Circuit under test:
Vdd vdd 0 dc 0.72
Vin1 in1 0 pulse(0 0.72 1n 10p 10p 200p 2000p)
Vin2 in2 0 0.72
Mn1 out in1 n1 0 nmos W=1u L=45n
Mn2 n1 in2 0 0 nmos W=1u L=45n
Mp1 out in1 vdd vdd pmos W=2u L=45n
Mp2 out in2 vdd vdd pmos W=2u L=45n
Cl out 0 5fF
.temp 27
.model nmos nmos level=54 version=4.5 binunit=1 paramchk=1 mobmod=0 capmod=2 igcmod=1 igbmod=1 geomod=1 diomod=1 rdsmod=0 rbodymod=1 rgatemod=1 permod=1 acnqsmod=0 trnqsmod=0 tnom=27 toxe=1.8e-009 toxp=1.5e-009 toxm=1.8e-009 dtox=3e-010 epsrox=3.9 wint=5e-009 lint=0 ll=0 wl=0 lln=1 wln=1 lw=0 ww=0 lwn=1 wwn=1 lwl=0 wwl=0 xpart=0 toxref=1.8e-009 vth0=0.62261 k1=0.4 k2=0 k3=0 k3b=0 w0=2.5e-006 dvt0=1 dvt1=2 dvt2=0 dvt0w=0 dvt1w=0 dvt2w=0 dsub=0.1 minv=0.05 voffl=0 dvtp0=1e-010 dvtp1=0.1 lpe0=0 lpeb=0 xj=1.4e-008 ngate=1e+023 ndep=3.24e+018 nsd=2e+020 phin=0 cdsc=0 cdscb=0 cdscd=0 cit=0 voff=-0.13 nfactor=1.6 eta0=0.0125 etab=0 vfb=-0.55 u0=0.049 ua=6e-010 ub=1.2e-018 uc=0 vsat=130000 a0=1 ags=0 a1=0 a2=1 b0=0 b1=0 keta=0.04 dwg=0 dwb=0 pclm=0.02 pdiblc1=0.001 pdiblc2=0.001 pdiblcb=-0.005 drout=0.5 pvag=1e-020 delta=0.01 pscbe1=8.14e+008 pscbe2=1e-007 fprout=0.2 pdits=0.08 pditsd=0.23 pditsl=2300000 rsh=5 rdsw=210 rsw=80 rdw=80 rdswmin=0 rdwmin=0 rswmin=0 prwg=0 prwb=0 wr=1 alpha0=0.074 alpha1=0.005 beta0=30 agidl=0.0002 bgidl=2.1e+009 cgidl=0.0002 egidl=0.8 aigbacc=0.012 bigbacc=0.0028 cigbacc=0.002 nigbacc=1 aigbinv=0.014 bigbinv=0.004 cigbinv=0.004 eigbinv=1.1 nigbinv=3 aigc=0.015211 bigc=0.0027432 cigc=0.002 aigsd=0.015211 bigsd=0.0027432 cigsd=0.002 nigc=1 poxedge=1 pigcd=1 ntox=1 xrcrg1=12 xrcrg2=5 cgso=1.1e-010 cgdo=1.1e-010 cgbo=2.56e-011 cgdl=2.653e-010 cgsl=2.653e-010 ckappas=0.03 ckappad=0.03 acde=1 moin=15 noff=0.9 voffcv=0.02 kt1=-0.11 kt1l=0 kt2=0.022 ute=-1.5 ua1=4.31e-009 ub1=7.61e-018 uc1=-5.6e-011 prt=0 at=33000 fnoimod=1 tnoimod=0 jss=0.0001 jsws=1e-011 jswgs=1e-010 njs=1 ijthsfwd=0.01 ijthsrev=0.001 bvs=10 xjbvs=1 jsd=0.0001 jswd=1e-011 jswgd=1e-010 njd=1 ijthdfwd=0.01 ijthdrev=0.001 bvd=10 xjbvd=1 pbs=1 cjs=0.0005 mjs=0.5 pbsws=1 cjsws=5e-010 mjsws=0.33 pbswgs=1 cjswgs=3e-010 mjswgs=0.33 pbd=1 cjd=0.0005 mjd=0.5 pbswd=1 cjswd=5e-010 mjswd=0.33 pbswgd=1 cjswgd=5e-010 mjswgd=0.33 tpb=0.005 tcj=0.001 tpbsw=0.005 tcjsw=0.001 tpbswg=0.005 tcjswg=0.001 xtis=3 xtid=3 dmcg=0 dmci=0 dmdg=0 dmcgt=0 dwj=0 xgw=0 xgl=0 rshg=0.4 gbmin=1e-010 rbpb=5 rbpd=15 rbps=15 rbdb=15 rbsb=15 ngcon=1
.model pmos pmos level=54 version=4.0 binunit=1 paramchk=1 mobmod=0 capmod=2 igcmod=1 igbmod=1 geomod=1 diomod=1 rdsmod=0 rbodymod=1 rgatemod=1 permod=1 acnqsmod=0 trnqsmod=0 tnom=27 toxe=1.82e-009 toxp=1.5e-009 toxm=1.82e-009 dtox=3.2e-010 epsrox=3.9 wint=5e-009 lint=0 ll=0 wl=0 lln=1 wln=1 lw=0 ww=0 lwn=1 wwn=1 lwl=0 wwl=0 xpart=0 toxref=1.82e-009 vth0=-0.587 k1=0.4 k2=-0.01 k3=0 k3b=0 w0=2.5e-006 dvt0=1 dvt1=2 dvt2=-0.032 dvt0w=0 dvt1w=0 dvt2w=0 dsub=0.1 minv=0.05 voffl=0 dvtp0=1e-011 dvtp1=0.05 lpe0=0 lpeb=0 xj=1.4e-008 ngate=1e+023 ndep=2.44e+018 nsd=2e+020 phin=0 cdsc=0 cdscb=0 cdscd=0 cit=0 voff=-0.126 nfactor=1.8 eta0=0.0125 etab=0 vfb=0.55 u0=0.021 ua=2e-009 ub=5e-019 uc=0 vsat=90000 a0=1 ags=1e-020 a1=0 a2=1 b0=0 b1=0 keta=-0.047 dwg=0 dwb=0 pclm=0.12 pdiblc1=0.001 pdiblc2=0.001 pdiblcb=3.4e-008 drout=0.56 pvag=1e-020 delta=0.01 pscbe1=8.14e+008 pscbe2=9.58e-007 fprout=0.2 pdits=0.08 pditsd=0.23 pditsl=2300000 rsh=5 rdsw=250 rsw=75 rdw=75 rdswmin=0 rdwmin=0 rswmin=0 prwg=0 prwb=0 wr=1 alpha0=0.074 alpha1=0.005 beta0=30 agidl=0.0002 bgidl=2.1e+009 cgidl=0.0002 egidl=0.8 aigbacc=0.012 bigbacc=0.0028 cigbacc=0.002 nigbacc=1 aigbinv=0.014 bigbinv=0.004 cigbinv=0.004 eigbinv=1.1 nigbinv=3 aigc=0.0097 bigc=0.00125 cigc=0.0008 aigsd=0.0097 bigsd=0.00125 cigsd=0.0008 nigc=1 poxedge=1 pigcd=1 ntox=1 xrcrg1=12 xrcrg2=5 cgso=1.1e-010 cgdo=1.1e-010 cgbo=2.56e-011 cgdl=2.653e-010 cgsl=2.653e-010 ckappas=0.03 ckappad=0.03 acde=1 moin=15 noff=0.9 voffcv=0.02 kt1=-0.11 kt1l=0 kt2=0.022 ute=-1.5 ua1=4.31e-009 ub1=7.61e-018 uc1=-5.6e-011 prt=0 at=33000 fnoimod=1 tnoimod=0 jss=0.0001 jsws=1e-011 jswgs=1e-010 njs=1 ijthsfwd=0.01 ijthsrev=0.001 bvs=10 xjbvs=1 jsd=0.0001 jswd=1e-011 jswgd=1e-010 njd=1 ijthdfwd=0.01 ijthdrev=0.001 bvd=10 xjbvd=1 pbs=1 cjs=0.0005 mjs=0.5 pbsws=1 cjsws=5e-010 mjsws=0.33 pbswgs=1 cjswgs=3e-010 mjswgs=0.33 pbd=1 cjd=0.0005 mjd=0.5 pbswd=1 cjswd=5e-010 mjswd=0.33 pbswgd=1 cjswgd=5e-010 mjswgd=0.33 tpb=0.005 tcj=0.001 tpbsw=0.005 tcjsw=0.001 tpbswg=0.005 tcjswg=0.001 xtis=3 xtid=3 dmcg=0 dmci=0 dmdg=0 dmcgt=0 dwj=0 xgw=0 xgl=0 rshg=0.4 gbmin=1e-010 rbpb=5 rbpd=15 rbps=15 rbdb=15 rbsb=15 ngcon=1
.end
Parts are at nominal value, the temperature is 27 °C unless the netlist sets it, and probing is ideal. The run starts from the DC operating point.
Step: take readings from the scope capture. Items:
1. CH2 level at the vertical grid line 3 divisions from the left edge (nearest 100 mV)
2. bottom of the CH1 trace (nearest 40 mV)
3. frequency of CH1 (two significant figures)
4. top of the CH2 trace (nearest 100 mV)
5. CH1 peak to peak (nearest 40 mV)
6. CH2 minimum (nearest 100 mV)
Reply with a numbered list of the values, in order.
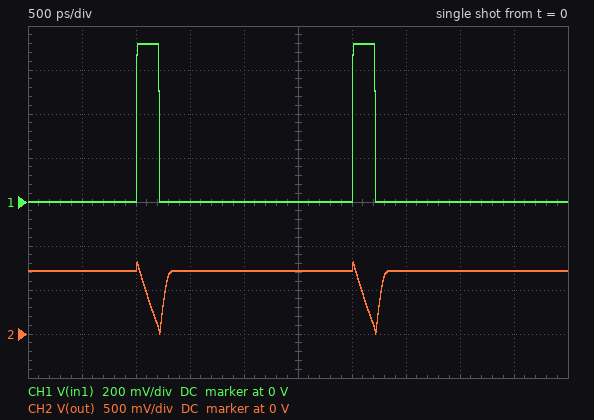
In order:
1. 700 mV
2. 0 V
3. 500 MHz
4. 800 mV
5. 720 mV
6. 0 V
